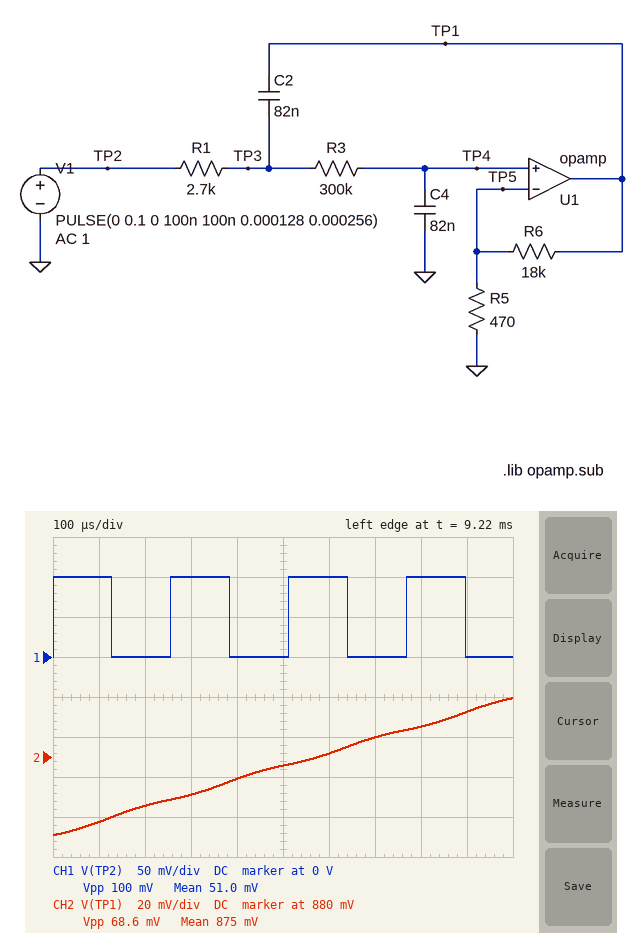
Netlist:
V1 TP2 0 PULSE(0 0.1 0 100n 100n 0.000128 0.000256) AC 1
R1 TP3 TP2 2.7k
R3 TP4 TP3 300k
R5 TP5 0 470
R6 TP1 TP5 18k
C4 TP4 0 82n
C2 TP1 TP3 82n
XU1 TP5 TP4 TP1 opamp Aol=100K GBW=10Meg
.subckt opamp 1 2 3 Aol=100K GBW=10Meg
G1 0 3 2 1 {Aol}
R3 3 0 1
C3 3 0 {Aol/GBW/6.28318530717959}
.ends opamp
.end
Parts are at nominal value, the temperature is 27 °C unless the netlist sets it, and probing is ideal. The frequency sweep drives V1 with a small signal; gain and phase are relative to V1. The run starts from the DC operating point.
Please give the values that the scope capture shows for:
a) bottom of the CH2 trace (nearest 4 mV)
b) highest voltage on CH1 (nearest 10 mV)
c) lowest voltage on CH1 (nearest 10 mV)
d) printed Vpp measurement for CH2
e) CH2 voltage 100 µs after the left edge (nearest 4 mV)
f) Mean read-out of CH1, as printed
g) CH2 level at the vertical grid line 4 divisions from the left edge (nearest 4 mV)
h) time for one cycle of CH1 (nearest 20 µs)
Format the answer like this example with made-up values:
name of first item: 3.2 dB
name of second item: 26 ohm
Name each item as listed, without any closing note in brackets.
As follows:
bottom of the CH2 trace: 840 mV
highest voltage on CH1: 100 mV
lowest voltage on CH1: 0 V
printed Vpp measurement for CH2: 68.6 mV
CH2 voltage 100 µs after the left edge: 848 mV
Mean read-out of CH1, as printed: 51.0 mV
CH2 level at the vertical grid line 4 divisions from the left edge: 868 mV
time for one cycle of CH1: 260 µs
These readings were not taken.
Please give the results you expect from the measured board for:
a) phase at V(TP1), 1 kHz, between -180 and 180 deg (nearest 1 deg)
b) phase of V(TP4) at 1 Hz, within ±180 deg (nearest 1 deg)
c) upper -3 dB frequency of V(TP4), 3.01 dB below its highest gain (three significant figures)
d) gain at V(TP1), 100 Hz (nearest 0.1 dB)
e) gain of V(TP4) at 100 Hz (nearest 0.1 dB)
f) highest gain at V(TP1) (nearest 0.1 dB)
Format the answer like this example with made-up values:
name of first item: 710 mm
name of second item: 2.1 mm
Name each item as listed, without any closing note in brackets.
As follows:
phase at V(TP1), 1 kHz, between -180 and 180 deg: -155 deg
phase of V(TP4) at 1 Hz, within ±180 deg: -6 deg
upper -3 dB frequency of V(TP4), 3.01 dB below its highest gain: 9.94 Hz
gain at V(TP1), 100 Hz: 11.6 dB
gain of V(TP4) at 100 Hz: -20.3 dB
highest gain at V(TP1): 31.9 dB
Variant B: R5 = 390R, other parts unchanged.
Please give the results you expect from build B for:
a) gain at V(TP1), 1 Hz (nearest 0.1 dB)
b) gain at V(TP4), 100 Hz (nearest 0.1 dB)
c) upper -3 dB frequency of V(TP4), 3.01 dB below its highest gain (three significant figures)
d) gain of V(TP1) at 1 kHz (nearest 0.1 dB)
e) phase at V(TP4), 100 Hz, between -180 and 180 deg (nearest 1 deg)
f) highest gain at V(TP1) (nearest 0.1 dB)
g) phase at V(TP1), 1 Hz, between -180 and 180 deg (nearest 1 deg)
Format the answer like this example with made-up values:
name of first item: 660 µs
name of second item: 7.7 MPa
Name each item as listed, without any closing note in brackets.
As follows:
gain at V(TP1), 1 Hz: 33.4 dB
gain at V(TP4), 100 Hz: -19.3 dB
upper -3 dB frequency of V(TP4), 3.01 dB below its highest gain: 11.2 Hz
gain of V(TP1) at 1 kHz: -13.9 dB
phase at V(TP4), 100 Hz, between -180 and 180 deg: -97 deg
highest gain at V(TP1): 33.5 dB
phase at V(TP1), 1 Hz, between -180 and 180 deg: -5 deg
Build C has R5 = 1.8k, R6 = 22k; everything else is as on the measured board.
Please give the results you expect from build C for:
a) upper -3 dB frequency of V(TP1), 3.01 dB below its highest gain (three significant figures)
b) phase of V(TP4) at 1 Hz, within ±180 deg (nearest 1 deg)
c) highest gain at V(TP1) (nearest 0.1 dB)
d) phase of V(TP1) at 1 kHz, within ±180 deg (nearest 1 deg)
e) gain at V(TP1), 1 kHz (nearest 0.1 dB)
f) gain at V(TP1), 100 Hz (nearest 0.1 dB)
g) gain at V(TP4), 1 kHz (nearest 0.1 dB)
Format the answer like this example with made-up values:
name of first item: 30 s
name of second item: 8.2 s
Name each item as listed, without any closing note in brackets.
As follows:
upper -3 dB frequency of V(TP1), 3.01 dB below its highest gain: 7.28 Hz
phase of V(TP4) at 1 Hz, within ±180 deg: -8 deg
highest gain at V(TP1): 22.4 dB
phase of V(TP1) at 1 kHz, within ±180 deg: -147 deg
gain at V(TP1), 1 kHz: -25.7 dB
gain at V(TP1), 100 Hz: -0.5 dB
gain at V(TP4), 1 kHz: -48.1 dB
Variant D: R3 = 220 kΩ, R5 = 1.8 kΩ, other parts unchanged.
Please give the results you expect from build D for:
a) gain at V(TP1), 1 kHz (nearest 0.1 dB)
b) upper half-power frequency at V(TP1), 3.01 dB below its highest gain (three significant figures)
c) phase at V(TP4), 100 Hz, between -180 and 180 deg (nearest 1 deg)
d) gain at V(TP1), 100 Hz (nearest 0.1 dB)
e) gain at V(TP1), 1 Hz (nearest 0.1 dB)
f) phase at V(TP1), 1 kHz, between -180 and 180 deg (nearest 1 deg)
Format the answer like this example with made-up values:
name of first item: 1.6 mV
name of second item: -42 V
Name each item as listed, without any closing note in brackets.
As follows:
gain at V(TP1), 1 kHz: -24.6 dB
upper half-power frequency at V(TP1), 3.01 dB below its highest gain: 10.1 Hz
phase at V(TP4), 100 Hz, between -180 and 180 deg: -93 deg
gain at V(TP1), 100 Hz: 0.7 dB
gain at V(TP1), 1 Hz: 20.8 dB
phase at V(TP1), 1 kHz, between -180 and 180 deg: -147 deg
